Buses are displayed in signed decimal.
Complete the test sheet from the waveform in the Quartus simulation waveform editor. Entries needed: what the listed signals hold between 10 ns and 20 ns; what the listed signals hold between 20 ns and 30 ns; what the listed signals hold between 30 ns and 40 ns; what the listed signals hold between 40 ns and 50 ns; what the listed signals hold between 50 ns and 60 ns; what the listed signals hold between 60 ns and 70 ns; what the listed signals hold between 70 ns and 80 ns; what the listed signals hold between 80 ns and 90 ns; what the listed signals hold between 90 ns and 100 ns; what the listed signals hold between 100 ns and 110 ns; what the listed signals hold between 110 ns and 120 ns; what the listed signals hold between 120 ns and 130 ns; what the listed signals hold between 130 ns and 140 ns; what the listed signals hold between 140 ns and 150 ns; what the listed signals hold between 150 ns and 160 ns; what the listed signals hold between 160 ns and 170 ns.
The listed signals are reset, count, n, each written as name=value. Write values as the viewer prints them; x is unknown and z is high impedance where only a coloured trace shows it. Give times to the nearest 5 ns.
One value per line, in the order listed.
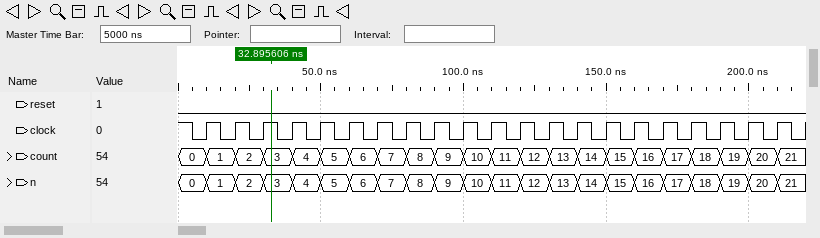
reset=0, count=1, n=1
reset=0, count=2, n=2
reset=0, count=3, n=3
reset=0, count=4, n=4
reset=0, count=5, n=5
reset=0, count=6, n=6
reset=0, count=7, n=7
reset=0, count=8, n=8
reset=0, count=9, n=9
reset=0, count=10, n=10
reset=0, count=11, n=11
reset=0, count=12, n=12
reset=0, count=13, n=13
reset=0, count=14, n=14
reset=0, count=15, n=15
reset=0, count=16, n=16
